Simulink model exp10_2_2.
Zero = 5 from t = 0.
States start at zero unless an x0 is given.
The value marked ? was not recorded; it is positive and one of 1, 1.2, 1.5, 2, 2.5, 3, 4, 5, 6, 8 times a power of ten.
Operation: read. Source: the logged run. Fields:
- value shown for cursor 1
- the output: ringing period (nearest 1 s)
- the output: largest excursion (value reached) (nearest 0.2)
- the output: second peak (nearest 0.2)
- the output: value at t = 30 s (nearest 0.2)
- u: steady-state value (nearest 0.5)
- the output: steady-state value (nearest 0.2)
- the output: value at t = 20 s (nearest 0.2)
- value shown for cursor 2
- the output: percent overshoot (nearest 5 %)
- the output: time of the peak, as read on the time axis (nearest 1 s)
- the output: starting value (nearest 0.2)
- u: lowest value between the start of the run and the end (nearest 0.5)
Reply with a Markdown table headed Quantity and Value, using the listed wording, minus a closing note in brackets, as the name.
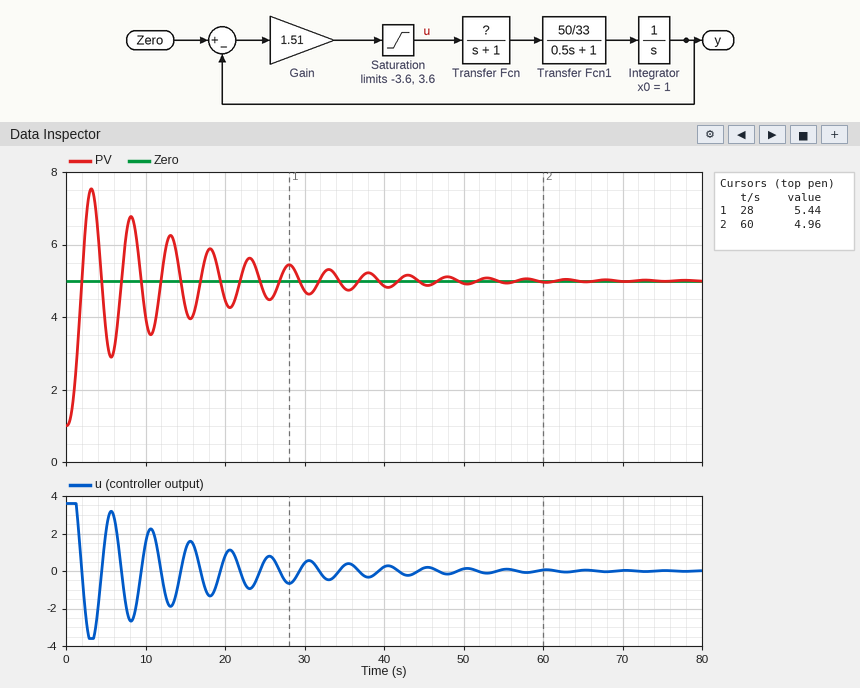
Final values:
| Quantity | Value |
|---|---|
| value shown for cursor 1 | 5.44 |
| the output: ringing period | 5 s |
| the output: largest excursion (value reached) | 7.6 |
| the output: second peak | 6.8 |
| the output: value at t = 30 s | 4.8 |
| u: steady-state value | 0.0 |
| the output: steady-state value | 5.0 |
| the output: value at t = 20 s | 4.4 |
| value shown for cursor 2 | 4.96 |
| the output: percent overshoot | 65 % |
| the output: time of the peak, as read on the time axis | 3 s |
| the output: starting value | 1.0 |
| u: lowest value between the start of the run and the end | -3.5 |
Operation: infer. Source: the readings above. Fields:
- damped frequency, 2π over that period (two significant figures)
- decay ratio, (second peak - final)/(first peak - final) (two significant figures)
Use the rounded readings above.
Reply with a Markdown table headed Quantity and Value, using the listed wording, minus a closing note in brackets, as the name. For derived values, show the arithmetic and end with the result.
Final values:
| Quantity | Value |
|---|---|
| damped frequency, 2π over that period | 2π / 5 = 1.3 rad/s |
| decay ratio, (second peak - final)/(first peak - final) | (6.8 - 5) / (7.6 - 5) = 0.69 |
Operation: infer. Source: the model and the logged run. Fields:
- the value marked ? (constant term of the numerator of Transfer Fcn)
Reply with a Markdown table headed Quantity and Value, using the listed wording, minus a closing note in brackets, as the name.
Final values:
| Quantity | Value |
|---|---|
| the value marked ? | 1 |
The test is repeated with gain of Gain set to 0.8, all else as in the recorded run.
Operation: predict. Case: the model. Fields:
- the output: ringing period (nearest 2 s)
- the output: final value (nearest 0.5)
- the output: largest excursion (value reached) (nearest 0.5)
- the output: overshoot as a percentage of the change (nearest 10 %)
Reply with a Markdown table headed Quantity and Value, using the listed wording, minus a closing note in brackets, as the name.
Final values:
| Quantity | Value |
|---|---|
| the output: ringing period | 6 s |
| the output: final value | 5.0 |
| the output: largest excursion (value reached) | 7.0 |
| the output: overshoot as a percentage of the change | 50 % |
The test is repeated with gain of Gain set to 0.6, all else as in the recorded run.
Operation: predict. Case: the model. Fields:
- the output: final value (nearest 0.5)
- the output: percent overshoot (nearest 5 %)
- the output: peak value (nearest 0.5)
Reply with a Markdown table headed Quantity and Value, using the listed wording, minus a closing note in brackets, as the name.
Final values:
| Quantity | Value |
|---|---|
| the output: final value | 5.0 |
| the output: percent overshoot | 35 % |
| the output: peak value | 6.5 |
